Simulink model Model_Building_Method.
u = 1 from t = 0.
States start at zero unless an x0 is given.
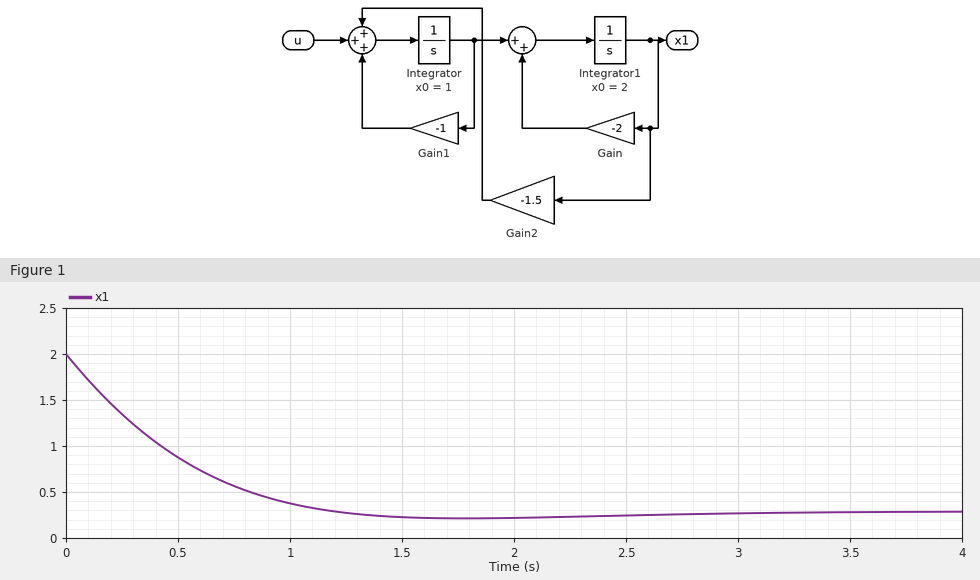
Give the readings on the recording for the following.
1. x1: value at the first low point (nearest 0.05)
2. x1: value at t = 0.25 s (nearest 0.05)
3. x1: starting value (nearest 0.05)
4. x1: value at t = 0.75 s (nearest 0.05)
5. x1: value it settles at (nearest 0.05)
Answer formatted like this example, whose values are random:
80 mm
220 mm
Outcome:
0.20
1.35
2.00
0.55
0.30
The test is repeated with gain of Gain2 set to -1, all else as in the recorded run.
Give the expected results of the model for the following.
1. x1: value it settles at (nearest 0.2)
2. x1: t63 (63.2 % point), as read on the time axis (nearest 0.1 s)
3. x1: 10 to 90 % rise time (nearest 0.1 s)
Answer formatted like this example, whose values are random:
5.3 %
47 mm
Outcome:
0.4
0.5 s
0.9 s
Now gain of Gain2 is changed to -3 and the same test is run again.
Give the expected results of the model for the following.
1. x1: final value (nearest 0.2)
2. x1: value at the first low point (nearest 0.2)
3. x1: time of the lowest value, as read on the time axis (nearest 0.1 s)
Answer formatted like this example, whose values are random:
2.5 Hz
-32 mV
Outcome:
0.2
0.0
1.4 s
